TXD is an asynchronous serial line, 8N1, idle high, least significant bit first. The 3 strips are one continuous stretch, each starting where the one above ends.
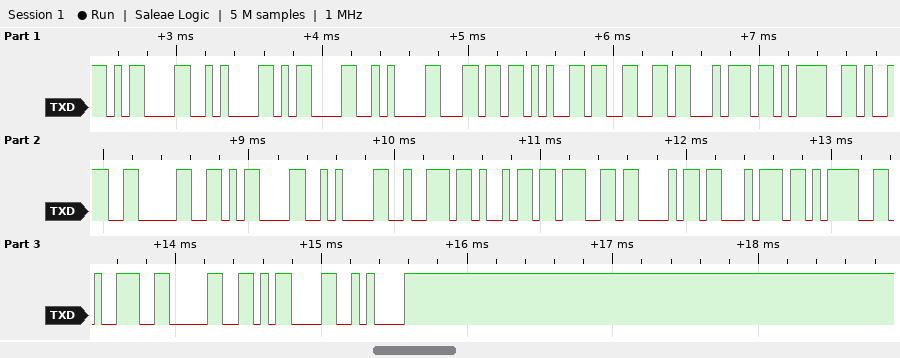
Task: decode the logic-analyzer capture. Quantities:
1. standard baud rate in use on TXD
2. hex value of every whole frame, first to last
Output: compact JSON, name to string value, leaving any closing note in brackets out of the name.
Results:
{"standard baud rate in use on TXD": "19200 baud", "hex value of every whole frame, first to last": "0D 0A 0D 0A 6C 65 66 74 3D 39 30 0D 0A 72 69 67 68 74 3D 39 30 0D 0A"}
